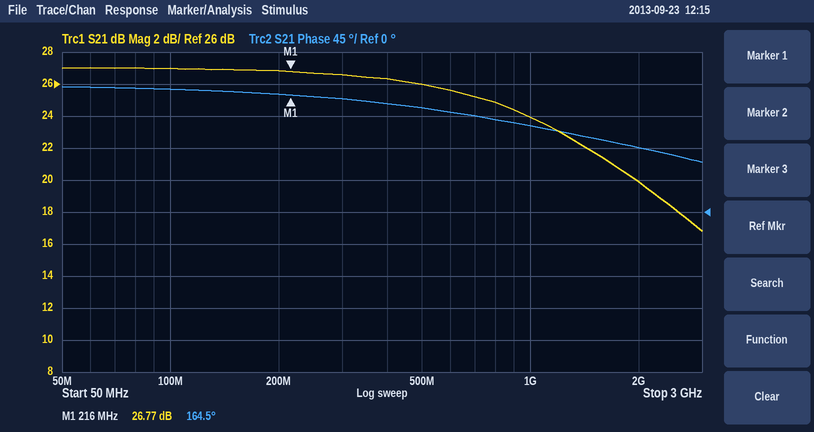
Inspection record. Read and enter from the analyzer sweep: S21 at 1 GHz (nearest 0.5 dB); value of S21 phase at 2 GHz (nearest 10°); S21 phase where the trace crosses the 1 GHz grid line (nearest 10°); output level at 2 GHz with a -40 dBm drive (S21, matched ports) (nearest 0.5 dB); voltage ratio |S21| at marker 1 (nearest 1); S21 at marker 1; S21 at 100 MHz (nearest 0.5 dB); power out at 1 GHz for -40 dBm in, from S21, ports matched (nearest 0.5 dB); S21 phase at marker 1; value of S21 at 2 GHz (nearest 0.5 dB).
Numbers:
24.0 dB
90°
120°
-20.0 dBm
22
26.77 dB
27.0 dB
-16.0 dBm
164.5°
20.0 dB
